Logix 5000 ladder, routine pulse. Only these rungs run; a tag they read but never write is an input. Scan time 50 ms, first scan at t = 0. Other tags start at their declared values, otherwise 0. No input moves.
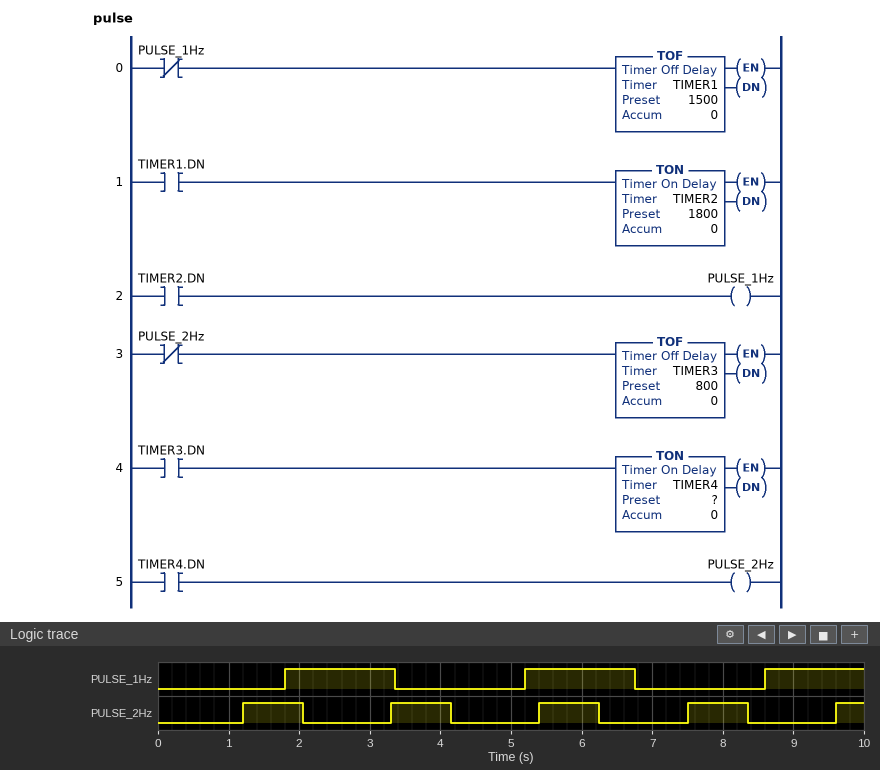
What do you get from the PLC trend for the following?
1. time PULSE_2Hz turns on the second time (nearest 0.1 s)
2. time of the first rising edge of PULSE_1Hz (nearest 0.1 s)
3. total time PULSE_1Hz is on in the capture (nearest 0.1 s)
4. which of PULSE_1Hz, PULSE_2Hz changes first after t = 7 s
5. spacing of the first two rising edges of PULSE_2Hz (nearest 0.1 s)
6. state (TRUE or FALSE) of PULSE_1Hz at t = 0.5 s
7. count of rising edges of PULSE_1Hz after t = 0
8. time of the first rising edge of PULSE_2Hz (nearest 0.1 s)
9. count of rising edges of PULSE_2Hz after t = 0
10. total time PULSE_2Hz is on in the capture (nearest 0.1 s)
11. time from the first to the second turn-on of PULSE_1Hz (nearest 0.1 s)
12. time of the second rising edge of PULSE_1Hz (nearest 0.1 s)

3.3 s
1.8 s
4.5 s
PULSE_2Hz
2.1 s
FALSE
3
1.2 s
5
3.8 s
3.4 s
5.2 s
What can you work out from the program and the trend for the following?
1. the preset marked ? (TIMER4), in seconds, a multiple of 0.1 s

1.2 s
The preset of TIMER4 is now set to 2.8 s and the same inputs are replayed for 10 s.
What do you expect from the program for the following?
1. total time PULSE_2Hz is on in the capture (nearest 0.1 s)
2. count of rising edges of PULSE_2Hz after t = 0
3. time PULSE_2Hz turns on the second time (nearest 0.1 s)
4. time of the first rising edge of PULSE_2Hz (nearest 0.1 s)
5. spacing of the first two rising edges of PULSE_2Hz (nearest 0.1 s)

1.7 s
2
6.5 s
2.8 s
3.7 s
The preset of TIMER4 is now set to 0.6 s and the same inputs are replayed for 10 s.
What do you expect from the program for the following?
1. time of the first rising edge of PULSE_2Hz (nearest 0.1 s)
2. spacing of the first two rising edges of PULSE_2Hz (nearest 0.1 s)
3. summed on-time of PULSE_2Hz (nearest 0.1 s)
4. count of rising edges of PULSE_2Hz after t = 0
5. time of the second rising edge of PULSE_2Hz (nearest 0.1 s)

0.6 s
1.5 s
5.5 s
7
2.1 s
